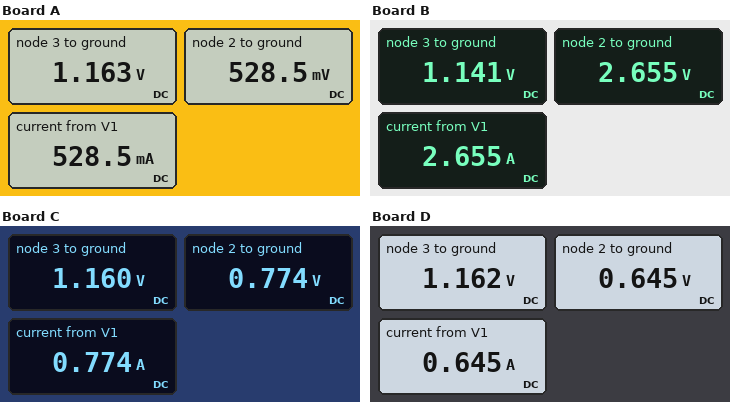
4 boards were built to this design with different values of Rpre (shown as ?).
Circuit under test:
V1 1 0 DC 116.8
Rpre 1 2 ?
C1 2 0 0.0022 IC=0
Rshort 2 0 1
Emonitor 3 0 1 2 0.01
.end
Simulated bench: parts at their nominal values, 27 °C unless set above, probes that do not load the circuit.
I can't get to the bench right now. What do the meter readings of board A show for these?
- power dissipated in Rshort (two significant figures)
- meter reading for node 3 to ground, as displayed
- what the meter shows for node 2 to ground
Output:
280 mW
1.163 V
528.5 mV
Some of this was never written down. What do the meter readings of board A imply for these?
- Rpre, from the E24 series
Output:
220 Ω
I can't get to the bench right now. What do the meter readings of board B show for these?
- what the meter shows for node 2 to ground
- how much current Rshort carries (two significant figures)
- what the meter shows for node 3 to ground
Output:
2.655 V
2.7 A
1.141 V
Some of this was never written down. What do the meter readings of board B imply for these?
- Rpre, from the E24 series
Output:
43 Ω
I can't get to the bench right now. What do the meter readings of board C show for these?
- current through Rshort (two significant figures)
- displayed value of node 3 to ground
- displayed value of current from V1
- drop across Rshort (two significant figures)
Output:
770 mA
1.160 V
0.774 A
770 mV
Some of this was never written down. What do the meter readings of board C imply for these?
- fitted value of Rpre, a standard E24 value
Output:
150 Ω
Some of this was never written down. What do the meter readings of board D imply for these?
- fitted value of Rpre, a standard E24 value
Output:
180 Ω
